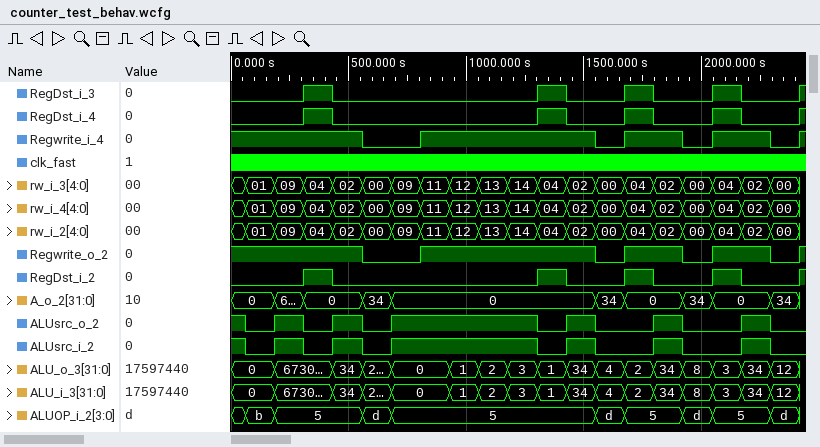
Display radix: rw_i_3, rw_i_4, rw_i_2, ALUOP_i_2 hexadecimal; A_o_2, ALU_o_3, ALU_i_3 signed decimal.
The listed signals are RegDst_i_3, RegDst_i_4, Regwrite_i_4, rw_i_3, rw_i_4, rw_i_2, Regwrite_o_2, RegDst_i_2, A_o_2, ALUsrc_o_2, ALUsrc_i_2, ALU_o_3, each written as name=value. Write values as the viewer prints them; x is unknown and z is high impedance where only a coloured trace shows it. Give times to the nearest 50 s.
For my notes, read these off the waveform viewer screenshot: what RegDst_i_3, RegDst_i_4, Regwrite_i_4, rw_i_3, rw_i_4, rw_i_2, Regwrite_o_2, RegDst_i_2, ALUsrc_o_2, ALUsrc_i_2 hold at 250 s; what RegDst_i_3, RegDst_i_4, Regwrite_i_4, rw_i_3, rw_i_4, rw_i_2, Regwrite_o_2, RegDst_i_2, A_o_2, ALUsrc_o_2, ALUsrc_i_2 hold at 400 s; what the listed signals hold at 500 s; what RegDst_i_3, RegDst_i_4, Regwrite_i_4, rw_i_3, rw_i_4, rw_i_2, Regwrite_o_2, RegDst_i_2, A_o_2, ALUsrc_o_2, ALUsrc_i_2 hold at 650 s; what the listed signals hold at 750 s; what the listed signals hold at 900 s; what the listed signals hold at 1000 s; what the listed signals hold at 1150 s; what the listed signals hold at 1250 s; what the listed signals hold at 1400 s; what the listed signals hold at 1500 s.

RegDst_i_3=0, RegDst_i_4=0, Regwrite_i_4=1, rw_i_3=09, rw_i_4=09, rw_i_2=09, Regwrite_o_2=1, RegDst_i_2=0, ALUsrc_o_2=1, ALUsrc_i_2=1
RegDst_i_3=1, RegDst_i_4=1, Regwrite_i_4=1, rw_i_3=04, rw_i_4=04, rw_i_2=04, Regwrite_o_2=1, RegDst_i_2=1, A_o_2=0, ALUsrc_o_2=0, ALUsrc_i_2=0
RegDst_i_3=0, RegDst_i_4=0, Regwrite_i_4=1, rw_i_3=02, rw_i_4=02, rw_i_2=02, Regwrite_o_2=1, RegDst_i_2=0, A_o_2=0, ALUsrc_o_2=1, ALUsrc_i_2=1, ALU_o_3=34
RegDst_i_3=0, RegDst_i_4=0, Regwrite_i_4=0, rw_i_3=00, rw_i_4=00, rw_i_2=00, Regwrite_o_2=0, RegDst_i_2=0, A_o_2=34, ALUsrc_o_2=0, ALUsrc_i_2=0
RegDst_i_3=0, RegDst_i_4=0, Regwrite_i_4=0, rw_i_3=09, rw_i_4=09, rw_i_2=09, Regwrite_o_2=0, RegDst_i_2=0, A_o_2=0, ALUsrc_o_2=1, ALUsrc_i_2=1, ALU_o_3=0
RegDst_i_3=0, RegDst_i_4=0, Regwrite_i_4=1, rw_i_3=11, rw_i_4=11, rw_i_2=11, Regwrite_o_2=1, RegDst_i_2=0, A_o_2=0, ALUsrc_o_2=1, ALUsrc_i_2=1, ALU_o_3=0
RegDst_i_3=0, RegDst_i_4=0, Regwrite_i_4=1, rw_i_3=12, rw_i_4=12, rw_i_2=12, Regwrite_o_2=1, RegDst_i_2=0, A_o_2=0, ALUsrc_o_2=1, ALUsrc_i_2=1, ALU_o_3=1
RegDst_i_3=0, RegDst_i_4=0, Regwrite_i_4=1, rw_i_3=13, rw_i_4=13, rw_i_2=13, Regwrite_o_2=1, RegDst_i_2=0, A_o_2=0, ALUsrc_o_2=1, ALUsrc_i_2=1, ALU_o_3=2
RegDst_i_3=0, RegDst_i_4=0, Regwrite_i_4=1, rw_i_3=14, rw_i_4=14, rw_i_2=14, Regwrite_o_2=1, RegDst_i_2=0, A_o_2=0, ALUsrc_o_2=1, ALUsrc_i_2=1, ALU_o_3=3
RegDst_i_3=1, RegDst_i_4=1, Regwrite_i_4=1, rw_i_3=04, rw_i_4=04, rw_i_2=04, Regwrite_o_2=1, RegDst_i_2=1, A_o_2=0, ALUsrc_o_2=0, ALUsrc_i_2=0, ALU_o_3=1
RegDst_i_3=0, RegDst_i_4=0, Regwrite_i_4=1, rw_i_3=02, rw_i_4=02, rw_i_2=02, Regwrite_o_2=1, RegDst_i_2=0, A_o_2=0, ALUsrc_o_2=1, ALUsrc_i_2=1, ALU_o_3=34
